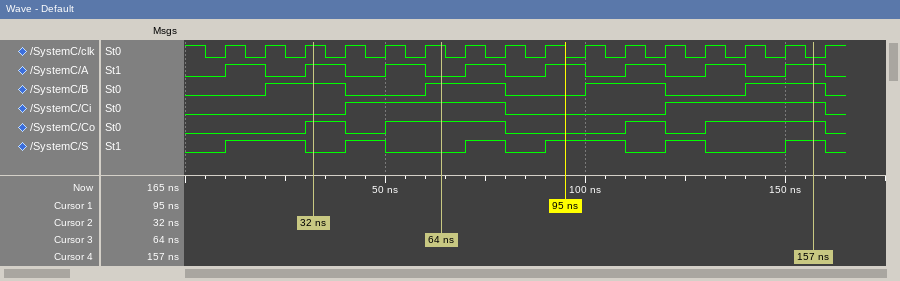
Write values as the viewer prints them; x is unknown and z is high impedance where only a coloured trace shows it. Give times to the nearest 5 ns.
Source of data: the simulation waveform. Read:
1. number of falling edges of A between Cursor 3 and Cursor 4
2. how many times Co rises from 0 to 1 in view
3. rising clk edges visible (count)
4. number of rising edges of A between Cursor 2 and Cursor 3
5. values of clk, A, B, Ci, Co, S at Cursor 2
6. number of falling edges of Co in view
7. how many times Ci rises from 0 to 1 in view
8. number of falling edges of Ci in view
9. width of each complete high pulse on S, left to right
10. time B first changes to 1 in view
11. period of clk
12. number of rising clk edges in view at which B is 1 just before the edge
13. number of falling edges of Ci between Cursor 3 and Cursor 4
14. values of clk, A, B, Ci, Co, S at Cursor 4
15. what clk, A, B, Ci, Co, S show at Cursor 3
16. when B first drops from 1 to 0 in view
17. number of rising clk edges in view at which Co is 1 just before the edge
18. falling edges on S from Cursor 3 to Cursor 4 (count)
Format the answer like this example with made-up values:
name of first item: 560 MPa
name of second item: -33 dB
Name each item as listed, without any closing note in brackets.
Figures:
number of falling edges of A between Cursor 3 and Cursor 4: 4
how many times Co rises from 0 to 1 in view: 4
rising clk edges visible: 16
number of rising edges of A between Cursor 2 and Cursor 3: 1
values of clk, A, B, Ci, Co, S at Cursor 2: clk=1, A=1, B=1, Ci=0, Co=1, S=0
number of falling edges of Co in view: 4
how many times Ci rises from 0 to 1 in view: 2
number of falling edges of Ci in view: 2
width of each complete high pulse on S, left to right: 20 ns, 10 ns, 10 ns, 20 ns, 10 ns, 10 ns
time B first changes to 1 in view: 20 ns
period of clk: 10 ns
number of rising clk edges in view at which B is 1 just before the edge: 8
number of falling edges of Ci between Cursor 3 and Cursor 4: 1
values of clk, A, B, Ci, Co, S at Cursor 4: clk=0, A=1, B=1, Ci=1, Co=1, S=1
what clk, A, B, Ci, Co, S show at Cursor 3: clk=1, A=0, B=1, Ci=1, Co=1, S=0
when B first drops from 1 to 0 in view: 40 ns
number of rising clk edges in view at which Co is 1 just before the edge: 8
falling edges on S from Cursor 3 to Cursor 4: 3
